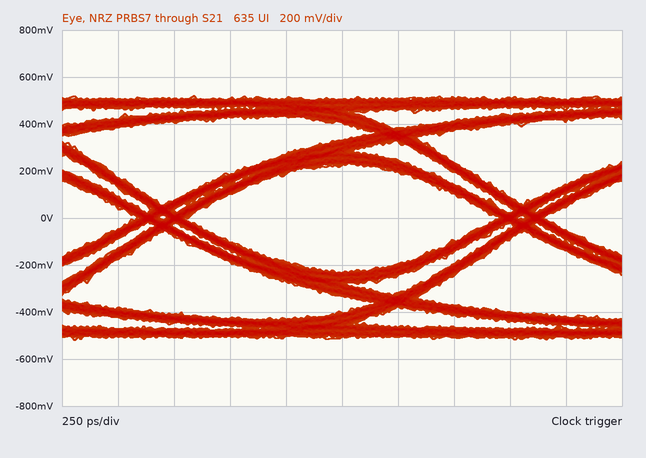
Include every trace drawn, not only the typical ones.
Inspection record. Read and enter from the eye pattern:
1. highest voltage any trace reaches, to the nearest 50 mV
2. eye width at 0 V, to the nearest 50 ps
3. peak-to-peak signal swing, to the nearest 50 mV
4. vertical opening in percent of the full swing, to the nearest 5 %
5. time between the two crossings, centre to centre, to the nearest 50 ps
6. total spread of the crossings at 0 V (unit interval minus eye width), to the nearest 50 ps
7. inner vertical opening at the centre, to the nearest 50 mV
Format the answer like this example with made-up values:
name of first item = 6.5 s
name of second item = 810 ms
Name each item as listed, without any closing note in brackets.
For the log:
highest voltage any trace reaches, to the nearest 50 mV = 500 mV
eye width at 0 V, to the nearest 50 ps = 1.40 ns
peak-to-peak signal swing, to the nearest 50 mV = 1.05 V
vertical opening in percent of the full swing, to the nearest 5 % = 45 %
time between the two crossings, centre to centre, to the nearest 50 ps = 1.60 ns
total spread of the crossings at 0 V (unit interval minus eye width), to the nearest 50 ps = 200 ps
inner vertical opening at the centre, to the nearest 50 mV = 450 mV
